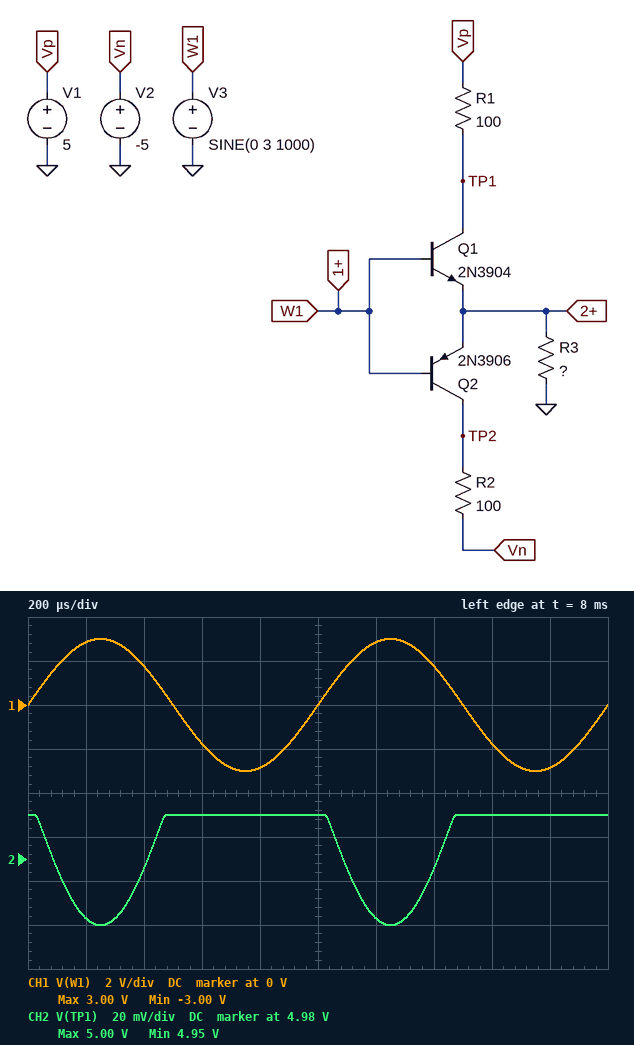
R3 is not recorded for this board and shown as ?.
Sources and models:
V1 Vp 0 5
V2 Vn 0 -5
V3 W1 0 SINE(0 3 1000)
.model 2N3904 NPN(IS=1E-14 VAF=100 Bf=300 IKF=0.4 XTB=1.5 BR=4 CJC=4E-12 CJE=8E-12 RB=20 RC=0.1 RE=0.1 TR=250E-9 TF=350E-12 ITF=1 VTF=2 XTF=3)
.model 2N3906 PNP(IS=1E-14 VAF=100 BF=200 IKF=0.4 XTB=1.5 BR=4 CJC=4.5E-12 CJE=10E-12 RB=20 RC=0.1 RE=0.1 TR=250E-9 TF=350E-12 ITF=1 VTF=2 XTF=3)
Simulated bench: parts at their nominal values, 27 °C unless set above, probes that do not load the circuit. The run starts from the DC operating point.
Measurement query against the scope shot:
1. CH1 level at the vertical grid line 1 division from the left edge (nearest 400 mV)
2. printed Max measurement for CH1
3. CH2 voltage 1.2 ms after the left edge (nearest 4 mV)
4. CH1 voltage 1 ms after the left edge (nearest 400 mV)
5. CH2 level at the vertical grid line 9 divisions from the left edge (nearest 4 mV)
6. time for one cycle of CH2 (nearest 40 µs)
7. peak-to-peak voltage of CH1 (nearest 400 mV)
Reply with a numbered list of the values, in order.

1. 2.8 V
2. 3.00 V
3. 4.952 V
4. 0 V
5. 5.000 V
6. 1.00 ms
7. 6.0 V
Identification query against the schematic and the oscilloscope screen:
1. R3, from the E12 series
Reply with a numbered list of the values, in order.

1. 4.7 kΩ
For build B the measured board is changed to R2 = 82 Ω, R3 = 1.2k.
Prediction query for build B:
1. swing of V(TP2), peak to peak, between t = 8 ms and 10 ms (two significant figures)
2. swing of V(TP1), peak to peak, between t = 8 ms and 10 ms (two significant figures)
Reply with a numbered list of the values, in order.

1. 160 mV
2. 190 mV
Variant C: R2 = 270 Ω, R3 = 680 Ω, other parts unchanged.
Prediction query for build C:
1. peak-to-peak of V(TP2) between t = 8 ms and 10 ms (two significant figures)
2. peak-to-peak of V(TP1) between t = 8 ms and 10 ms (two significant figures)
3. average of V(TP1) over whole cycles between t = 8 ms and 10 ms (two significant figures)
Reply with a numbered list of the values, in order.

1. 910 mV
2. 340 mV
3. 4.9 V
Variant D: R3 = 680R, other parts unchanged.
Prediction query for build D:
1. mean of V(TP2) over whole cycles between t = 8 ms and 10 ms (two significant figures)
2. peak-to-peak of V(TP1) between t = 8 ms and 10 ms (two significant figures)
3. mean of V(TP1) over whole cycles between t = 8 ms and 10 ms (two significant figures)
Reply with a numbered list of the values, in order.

1. -4.9 V
2. 340 mV
3. 4.9 V
